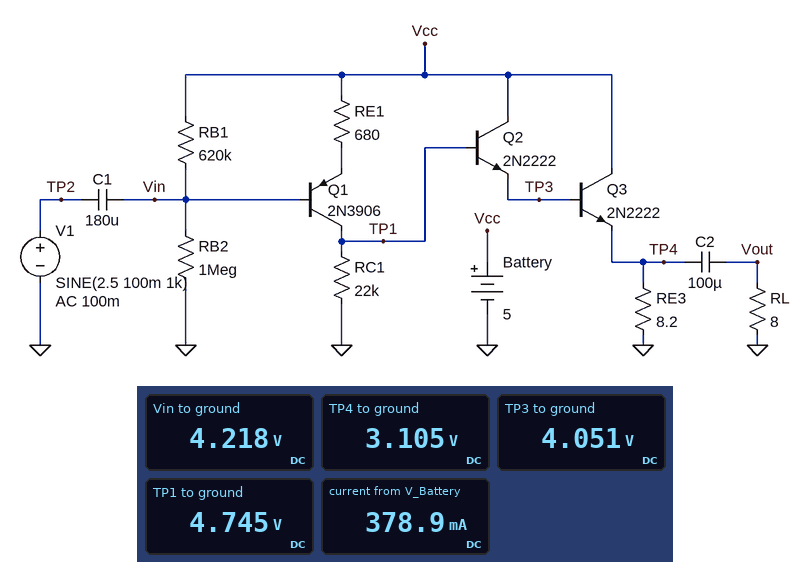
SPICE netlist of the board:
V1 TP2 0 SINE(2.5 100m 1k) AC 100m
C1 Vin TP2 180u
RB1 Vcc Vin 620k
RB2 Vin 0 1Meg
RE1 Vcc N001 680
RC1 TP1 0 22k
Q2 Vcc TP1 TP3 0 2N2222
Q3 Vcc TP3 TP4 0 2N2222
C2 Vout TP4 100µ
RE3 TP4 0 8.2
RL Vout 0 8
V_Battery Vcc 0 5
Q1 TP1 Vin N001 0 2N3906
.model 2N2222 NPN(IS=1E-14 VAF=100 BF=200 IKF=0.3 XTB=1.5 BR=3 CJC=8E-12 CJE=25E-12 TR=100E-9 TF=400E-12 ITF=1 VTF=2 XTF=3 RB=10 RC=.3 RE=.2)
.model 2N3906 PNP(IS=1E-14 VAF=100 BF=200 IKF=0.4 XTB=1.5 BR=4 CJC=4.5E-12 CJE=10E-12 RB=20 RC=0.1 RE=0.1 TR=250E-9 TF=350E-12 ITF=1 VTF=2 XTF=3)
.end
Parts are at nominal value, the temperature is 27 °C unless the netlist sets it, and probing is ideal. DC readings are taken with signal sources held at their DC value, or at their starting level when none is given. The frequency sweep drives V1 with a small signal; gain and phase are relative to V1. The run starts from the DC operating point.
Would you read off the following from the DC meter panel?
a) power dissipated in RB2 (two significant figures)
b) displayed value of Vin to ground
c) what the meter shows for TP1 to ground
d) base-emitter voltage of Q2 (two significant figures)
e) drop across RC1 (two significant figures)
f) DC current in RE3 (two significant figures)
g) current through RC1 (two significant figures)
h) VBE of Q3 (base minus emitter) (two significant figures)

18 µW
4.218 V
4.745 V
690 mV
4.7 V
380 mA
220 µA
950 mV
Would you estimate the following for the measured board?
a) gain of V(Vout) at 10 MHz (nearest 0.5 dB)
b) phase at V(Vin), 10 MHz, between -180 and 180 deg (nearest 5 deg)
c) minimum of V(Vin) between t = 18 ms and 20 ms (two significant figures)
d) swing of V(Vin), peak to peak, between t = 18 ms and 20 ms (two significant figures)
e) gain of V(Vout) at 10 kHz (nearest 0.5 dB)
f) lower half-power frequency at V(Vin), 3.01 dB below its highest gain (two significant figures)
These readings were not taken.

-2.5 dB
0 deg
4.1 V
200 mV
15.5 dB
500 mHz
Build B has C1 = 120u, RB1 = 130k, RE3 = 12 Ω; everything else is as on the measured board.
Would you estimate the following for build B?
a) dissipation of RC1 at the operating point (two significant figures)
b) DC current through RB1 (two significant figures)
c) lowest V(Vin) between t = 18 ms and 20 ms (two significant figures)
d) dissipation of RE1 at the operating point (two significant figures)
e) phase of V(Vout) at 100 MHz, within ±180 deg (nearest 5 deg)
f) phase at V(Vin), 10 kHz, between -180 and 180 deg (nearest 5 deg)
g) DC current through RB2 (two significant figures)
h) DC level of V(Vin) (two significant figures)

8.0 µW
4.3 µA
4.3 V
250 nW
85 deg
0 deg
4.4 µA
4.4 V
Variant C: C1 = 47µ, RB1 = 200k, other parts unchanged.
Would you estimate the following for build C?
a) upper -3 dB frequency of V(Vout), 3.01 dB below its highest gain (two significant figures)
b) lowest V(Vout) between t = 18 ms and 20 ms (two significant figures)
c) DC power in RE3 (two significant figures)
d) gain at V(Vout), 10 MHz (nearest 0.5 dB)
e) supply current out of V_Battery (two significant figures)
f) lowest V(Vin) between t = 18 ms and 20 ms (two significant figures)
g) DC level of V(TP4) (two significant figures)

820 kHz
-990 mV
320 mW
1.0 dB
200 mA
4.2 V
1.6 V
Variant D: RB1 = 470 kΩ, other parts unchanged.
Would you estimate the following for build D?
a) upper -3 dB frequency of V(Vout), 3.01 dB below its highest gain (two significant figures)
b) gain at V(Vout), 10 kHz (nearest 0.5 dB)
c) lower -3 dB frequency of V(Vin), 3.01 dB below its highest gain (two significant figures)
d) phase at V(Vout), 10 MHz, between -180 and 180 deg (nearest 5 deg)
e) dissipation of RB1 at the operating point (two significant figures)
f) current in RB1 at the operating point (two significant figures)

340 kHz
17.0 dB
450 mHz
0 deg
1.3 µW
1.7 µA
